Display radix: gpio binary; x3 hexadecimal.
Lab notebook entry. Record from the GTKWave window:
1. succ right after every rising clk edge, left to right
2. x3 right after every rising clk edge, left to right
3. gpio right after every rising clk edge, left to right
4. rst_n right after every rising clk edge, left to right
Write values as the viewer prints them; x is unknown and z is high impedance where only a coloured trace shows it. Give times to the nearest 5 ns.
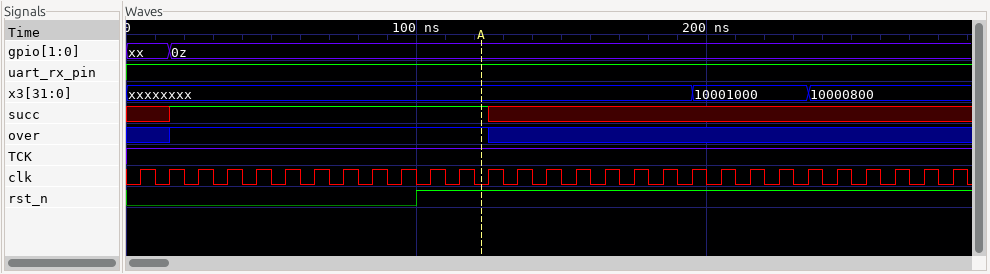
x 1 1 1 1 1 1 1 1 1 1 1 x x x x x x x x x x x x x x x x x
xxxxxxxx, xxxxxxxx, xxxxxxxx, xxxxxxxx, xxxxxxxx, xxxxxxxx, xxxxxxxx, xxxxxxxx, xxxxxxxx, xxxxxxxx, xxxxxxxx, xxxxxxxx, xxxxxxxx, xxxxxxxx, xxxxxxxx, xxxxxxxx, xxxxxxxx, xxxxxxxx, xxxxxxxx, 10001000, 10001000, 10001000, 10001000, 10000800, 10000800, 10000800, 10000800, 10000800, 10000800
xx, 0z, 0z, 0z, 0z, 0z, 0z, 0z, 0z, 0z, 0z, 0z, 0z, 0z, 0z, 0z, 0z, 0z, 0z, 0z, 0z, 0z, 0z, 0z, 0z, 0z, 0z, 0z, 0z
0 0 0 0 0 0 0 0 0 0 1 1 1 1 1 1 1 1 1 1 1 1 1 1 1 1 1 1 1
